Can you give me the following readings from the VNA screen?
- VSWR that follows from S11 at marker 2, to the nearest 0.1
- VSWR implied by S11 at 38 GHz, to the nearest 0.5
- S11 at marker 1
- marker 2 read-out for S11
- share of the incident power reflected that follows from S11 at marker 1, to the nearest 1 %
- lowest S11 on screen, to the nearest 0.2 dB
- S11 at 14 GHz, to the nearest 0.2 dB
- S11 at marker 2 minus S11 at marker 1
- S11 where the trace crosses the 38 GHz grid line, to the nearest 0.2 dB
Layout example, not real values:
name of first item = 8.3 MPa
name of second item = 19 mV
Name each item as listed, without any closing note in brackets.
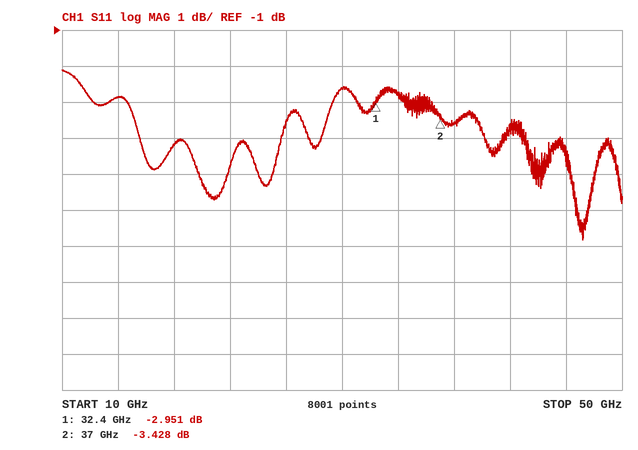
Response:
VSWR that follows from S11 at marker 2, to the nearest 0.1 = 5.1
VSWR implied by S11 at 38 GHz, to the nearest 0.5 = 5.0
S11 at marker 1 = -2.951 dB
marker 2 read-out for S11 = -3.428 dB
share of the incident power reflected that follows from S11 at marker 1, to the nearest 1 % = 51 %
lowest S11 on screen, to the nearest 0.2 dB = -6.8 dB
S11 at 14 GHz, to the nearest 0.2 dB = -2.8 dB
S11 at marker 2 minus S11 at marker 1 = -0.477 dB
S11 where the trace crosses the 38 GHz grid line, to the nearest 0.2 dB = -3.6 dB
